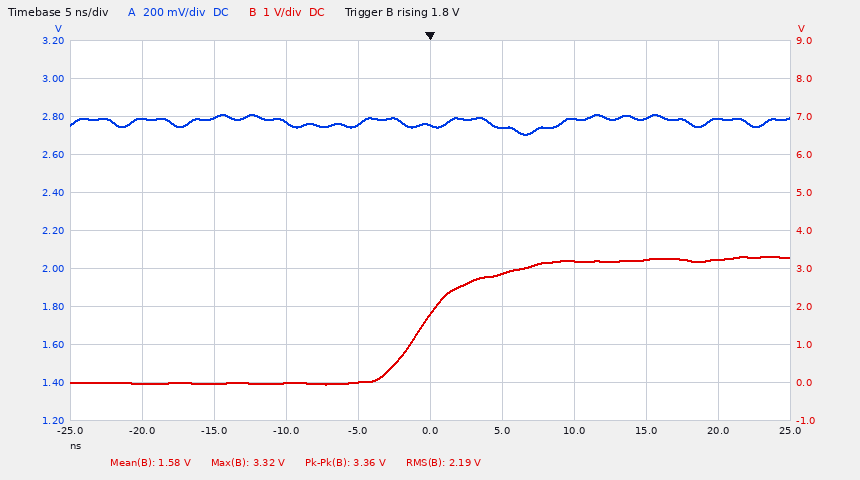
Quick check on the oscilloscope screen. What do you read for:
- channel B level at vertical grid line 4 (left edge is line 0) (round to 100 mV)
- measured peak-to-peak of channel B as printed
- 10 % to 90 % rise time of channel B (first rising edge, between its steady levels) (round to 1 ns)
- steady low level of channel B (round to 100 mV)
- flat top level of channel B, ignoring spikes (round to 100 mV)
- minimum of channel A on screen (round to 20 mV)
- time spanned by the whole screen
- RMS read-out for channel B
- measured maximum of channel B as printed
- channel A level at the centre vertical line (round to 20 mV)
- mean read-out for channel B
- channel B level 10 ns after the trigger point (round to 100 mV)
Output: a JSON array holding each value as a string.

["0.0 V", "3.36 V", "8 ns", "0.0 V", "3.2 V", "2.70 V", "50 ns", "2.19 V", "3.32 V", "2.76 V", "1.58 V", "3.2 V"]
